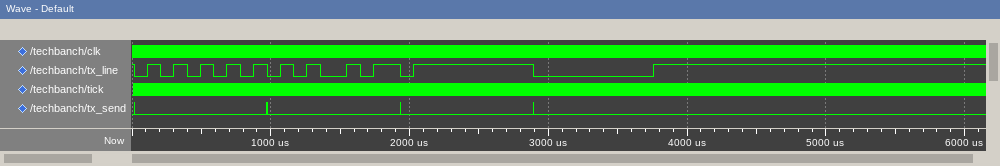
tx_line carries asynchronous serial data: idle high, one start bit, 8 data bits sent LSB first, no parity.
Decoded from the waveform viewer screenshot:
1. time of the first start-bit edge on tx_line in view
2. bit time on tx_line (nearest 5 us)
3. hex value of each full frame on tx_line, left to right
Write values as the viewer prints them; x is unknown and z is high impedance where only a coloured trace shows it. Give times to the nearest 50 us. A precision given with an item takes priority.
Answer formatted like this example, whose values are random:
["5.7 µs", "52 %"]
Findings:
["0 us", "95 us", "55, A5, FF, 00"]
